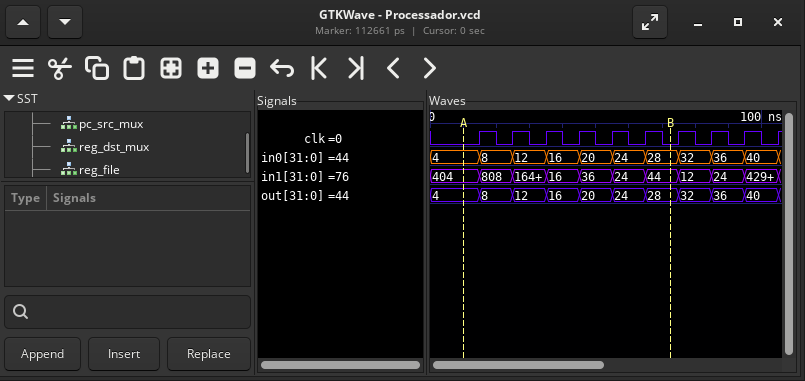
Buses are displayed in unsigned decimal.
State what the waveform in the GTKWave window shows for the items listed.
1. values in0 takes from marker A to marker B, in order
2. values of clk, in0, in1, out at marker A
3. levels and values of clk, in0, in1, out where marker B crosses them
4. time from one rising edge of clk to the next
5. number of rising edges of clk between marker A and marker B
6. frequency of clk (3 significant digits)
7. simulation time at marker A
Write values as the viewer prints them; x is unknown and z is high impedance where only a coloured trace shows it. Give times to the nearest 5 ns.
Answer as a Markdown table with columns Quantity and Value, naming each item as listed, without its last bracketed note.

| Quantity | Value |
|---|---|
| values in0 takes from marker A to marker B, in order | 4, 8, 12, 16, 20, 24, 28 |
| values of clk, in0, in1, out at marker A | clk=0, in0=4, in1=404, out=4 |
| levels and values of clk, in0, in1, out where marker B crosses them | clk=0, in0=28, in1=44, out=28 |
| time from one rising edge of clk to the next | 10 ns |
| number of rising edges of clk between marker A and marker B | 6 |
| frequency of clk | 100 MHz |
| simulation time at marker A | 10 ns |
